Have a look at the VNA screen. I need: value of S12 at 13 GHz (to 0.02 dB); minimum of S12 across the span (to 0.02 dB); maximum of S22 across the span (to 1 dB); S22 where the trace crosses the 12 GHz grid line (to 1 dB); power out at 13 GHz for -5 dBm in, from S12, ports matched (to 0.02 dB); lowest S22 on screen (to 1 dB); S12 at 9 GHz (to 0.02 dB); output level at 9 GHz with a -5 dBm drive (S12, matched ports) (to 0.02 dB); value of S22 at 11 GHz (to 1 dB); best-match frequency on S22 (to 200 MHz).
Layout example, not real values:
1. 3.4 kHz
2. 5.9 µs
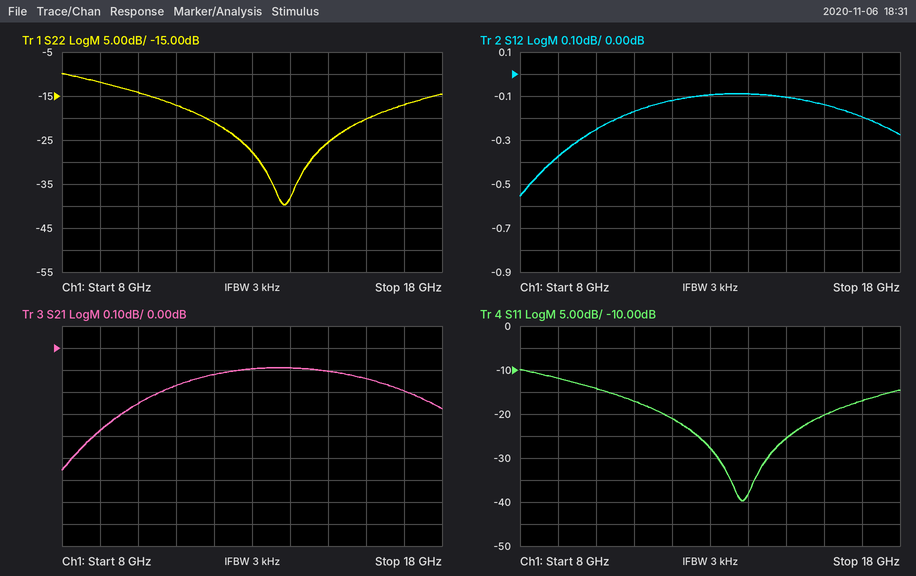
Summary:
1. -0.10 dB
2. -0.56 dB
3. -10 dB
4. -21 dB
5. -5.10 dBm
6. -40 dB
7. -0.38 dB
8. -5.38 dBm
9. -17 dB
10. 13.8 GHz
